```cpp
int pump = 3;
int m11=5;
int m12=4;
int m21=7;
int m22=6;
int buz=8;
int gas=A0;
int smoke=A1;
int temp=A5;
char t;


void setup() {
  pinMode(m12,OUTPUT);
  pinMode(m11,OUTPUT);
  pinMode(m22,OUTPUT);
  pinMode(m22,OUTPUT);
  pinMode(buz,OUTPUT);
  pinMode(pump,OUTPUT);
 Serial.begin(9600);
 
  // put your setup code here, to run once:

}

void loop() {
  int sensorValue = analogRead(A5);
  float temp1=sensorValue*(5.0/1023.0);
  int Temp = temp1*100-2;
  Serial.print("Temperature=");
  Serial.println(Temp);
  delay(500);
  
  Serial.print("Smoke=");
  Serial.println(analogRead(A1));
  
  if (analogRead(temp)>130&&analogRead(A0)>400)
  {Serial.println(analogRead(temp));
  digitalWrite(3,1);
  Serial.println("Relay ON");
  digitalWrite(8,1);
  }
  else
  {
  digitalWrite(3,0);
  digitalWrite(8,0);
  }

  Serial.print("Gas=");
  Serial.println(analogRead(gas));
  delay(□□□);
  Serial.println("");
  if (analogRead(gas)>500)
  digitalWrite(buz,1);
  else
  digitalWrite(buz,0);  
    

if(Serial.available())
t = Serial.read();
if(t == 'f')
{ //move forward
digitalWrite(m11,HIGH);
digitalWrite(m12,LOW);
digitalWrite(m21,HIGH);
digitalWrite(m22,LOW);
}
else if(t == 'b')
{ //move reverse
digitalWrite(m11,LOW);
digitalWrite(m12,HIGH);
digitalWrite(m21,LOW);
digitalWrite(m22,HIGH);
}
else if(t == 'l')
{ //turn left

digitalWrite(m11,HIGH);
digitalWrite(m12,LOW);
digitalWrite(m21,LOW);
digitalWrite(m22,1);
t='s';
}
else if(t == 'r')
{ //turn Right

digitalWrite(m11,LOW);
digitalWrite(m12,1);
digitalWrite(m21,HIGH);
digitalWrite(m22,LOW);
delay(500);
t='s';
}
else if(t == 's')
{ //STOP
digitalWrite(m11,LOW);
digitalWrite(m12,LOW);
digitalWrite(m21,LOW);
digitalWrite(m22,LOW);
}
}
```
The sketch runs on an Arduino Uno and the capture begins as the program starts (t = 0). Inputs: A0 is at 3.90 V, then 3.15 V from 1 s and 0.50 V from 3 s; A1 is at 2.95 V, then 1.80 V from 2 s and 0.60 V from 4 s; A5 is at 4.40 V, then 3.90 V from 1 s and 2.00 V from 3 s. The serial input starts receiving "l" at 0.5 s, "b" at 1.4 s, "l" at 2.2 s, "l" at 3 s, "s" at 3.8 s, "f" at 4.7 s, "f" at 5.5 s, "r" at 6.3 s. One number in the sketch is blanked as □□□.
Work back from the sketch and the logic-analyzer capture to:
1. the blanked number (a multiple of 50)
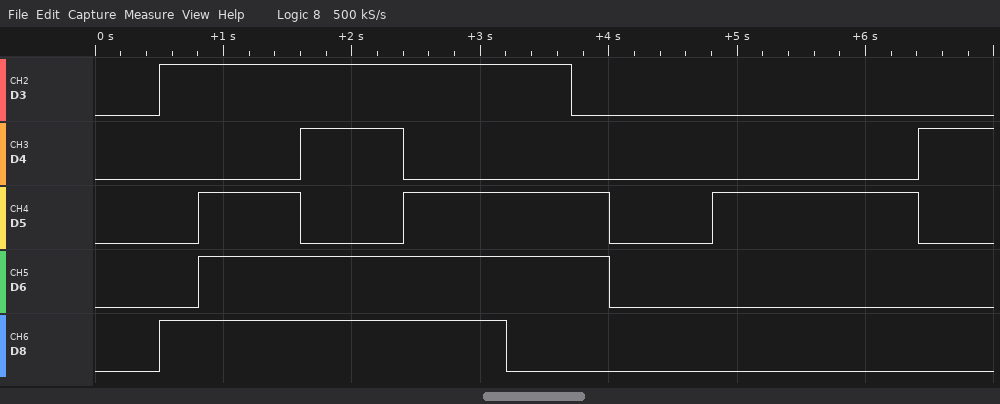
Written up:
300
